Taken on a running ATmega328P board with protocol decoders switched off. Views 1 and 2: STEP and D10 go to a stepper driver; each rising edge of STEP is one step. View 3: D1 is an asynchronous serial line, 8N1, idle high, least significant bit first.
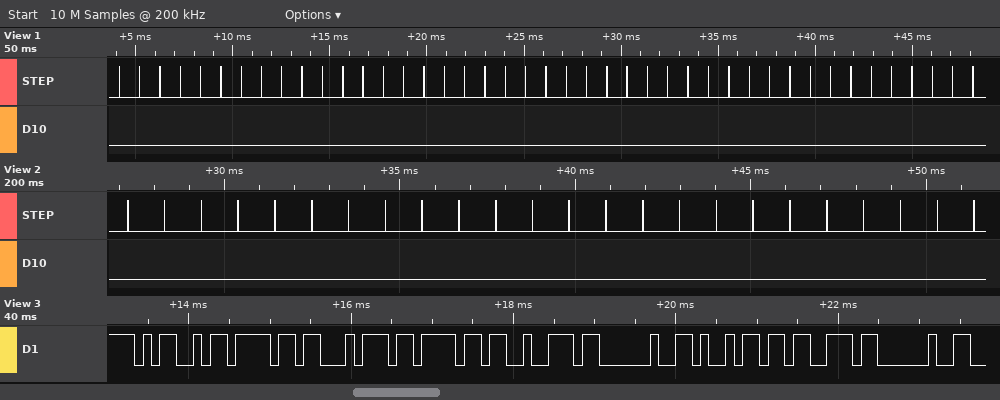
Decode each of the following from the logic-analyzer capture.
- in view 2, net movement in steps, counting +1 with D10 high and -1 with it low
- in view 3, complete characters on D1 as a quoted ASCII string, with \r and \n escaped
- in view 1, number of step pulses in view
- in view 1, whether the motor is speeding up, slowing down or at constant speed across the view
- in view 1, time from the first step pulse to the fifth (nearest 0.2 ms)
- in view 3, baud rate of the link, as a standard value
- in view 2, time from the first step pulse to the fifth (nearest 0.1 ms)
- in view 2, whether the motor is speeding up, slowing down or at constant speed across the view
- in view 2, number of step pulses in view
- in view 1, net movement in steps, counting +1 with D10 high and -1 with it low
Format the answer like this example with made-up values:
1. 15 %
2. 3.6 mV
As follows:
1. -24
2. "Motor is "
3. 43
4. constant speed
5. 4.2 ms
6. 9600 baud
7. 4.2 ms
8. constant speed
9. 24
10. -43
